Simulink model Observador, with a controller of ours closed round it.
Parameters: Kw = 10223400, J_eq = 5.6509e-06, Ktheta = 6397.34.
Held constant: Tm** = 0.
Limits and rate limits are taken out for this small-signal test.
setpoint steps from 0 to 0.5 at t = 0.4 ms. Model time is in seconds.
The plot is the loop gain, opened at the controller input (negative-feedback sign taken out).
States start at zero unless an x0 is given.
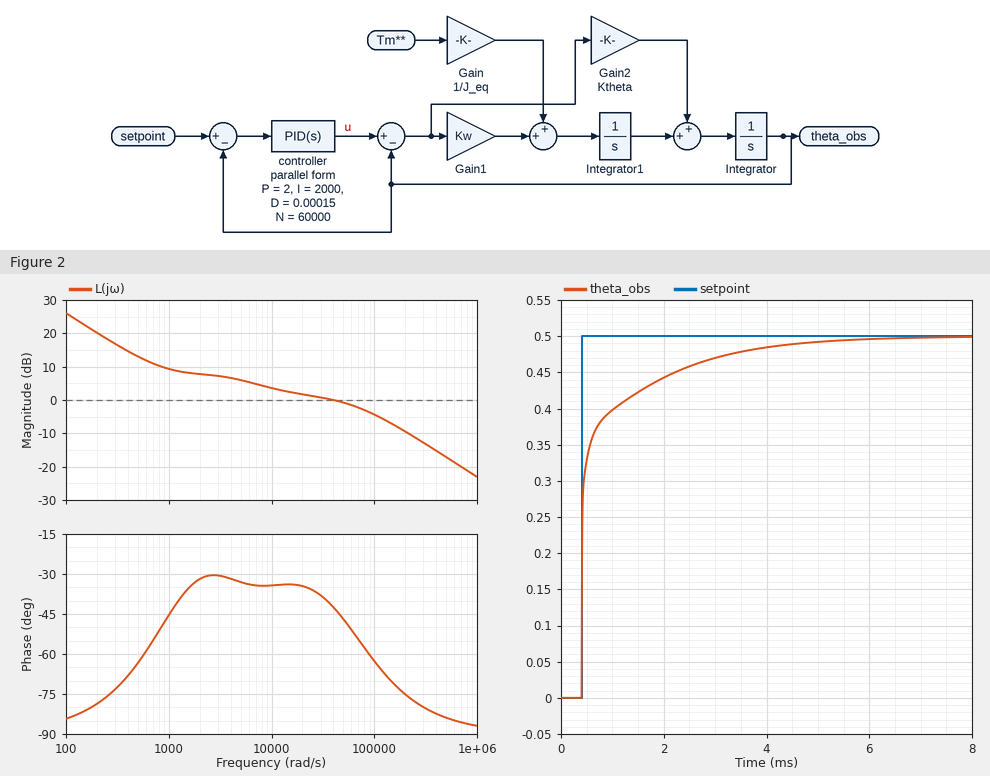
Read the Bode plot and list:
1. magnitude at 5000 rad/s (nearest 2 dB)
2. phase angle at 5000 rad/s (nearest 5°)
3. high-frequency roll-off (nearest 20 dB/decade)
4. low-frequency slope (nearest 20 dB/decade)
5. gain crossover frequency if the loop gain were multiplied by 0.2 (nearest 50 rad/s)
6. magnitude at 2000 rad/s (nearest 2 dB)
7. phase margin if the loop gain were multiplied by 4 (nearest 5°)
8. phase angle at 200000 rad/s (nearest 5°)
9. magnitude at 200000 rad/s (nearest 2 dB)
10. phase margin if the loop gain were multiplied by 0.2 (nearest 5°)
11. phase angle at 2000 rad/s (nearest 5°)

6 dB
-35°
-20 dB/decade
-20 dB/decade
450 rad/s
8 dB
100°
-75°
-10 dB
115°
-30°
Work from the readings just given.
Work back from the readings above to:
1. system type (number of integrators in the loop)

1
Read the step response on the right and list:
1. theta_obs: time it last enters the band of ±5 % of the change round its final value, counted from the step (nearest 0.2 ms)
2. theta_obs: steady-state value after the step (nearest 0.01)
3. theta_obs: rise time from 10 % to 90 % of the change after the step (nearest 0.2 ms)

2.8 ms
0.50
1.8 ms
